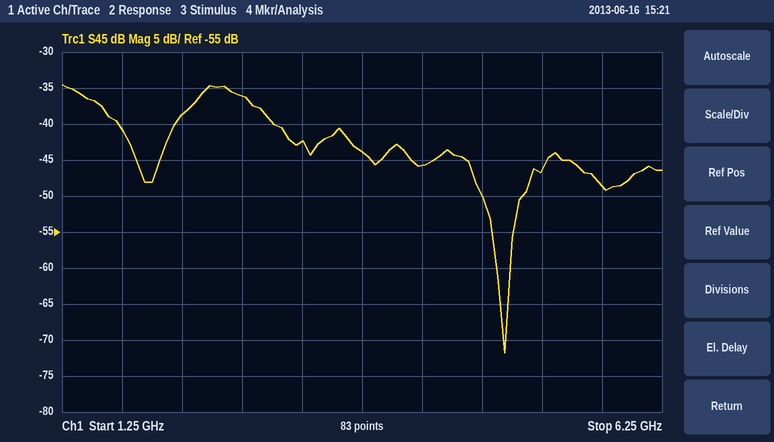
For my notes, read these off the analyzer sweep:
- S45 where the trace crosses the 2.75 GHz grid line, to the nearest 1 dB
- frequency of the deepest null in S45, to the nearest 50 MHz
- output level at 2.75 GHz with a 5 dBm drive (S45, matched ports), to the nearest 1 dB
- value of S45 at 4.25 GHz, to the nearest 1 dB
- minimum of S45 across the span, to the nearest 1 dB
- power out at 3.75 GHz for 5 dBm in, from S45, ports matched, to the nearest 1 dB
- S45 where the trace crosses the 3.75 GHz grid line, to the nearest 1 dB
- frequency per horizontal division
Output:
-36 dB
4.95 GHz
-31 dBm
-46 dB
-72 dB
-39 dBm
-44 dB
500 MHz
